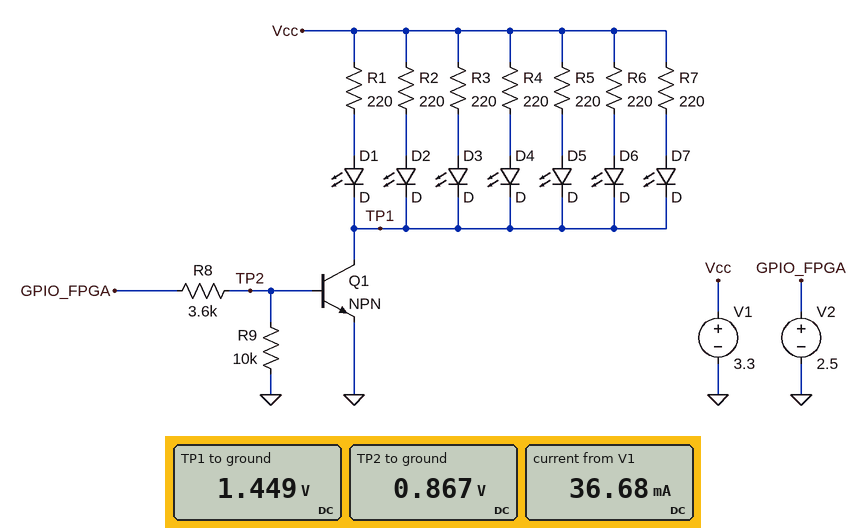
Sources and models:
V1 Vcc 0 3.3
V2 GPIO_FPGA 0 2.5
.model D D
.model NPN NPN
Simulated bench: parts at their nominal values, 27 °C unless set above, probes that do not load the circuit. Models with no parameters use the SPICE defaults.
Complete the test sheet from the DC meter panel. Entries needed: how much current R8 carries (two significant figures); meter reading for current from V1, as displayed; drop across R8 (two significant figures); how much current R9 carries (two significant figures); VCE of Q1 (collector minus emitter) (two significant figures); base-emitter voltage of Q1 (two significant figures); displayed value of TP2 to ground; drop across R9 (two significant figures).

450 µA
36.68 mA
1.6 V
87 µA
1.4 V
870 mV
0.867 V
870 mV
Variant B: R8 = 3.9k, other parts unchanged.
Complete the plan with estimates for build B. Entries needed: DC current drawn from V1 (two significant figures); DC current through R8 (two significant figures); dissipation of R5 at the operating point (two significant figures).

33 mA
420 µA
5.0 mW
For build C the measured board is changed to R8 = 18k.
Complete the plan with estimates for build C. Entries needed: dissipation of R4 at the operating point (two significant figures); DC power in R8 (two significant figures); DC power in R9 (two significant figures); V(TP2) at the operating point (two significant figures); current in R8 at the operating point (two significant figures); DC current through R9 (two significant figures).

12 µW
160 µW
62 µW
790 mV
95 µA
79 µA
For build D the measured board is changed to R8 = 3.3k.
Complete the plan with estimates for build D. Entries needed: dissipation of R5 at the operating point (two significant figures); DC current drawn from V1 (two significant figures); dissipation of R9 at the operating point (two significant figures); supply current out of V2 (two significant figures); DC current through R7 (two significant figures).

7.4 mW
41 mA
76 µW
490 µA
5.8 mA
